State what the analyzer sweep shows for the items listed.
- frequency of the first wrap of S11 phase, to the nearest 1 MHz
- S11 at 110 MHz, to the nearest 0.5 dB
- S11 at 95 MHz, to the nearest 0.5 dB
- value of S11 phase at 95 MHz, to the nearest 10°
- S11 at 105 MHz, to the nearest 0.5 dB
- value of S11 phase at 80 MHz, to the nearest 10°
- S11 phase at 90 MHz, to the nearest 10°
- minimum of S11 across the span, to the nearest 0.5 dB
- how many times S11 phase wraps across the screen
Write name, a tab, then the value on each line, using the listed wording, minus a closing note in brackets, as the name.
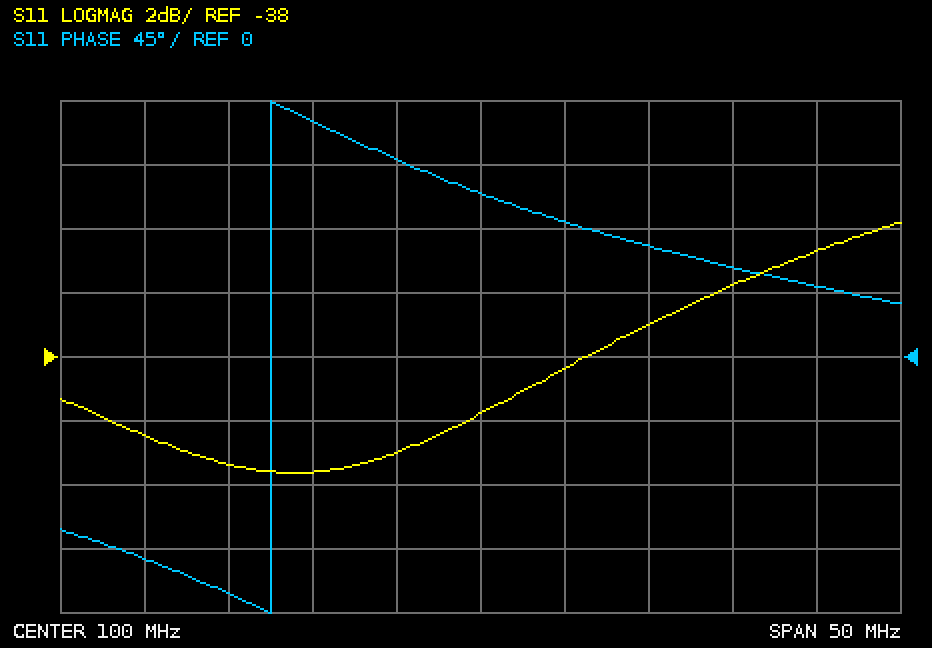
frequency of the first wrap of S11 phase, to the nearest 1 MHz	88 MHz
S11 at 110 MHz, to the nearest 0.5 dB	-37.0 dB
S11 at 95 MHz, to the nearest 0.5 dB	-41.0 dB
value of S11 phase at 95 MHz, to the nearest 10°	140°
S11 at 105 MHz, to the nearest 0.5 dB	-38.5 dB
value of S11 phase at 80 MHz, to the nearest 10°	-140°
S11 phase at 90 MHz, to the nearest 10°	170°
minimum of S11 across the span, to the nearest 0.5 dB	-41.5 dB
how many times S11 phase wraps across the screen	1
